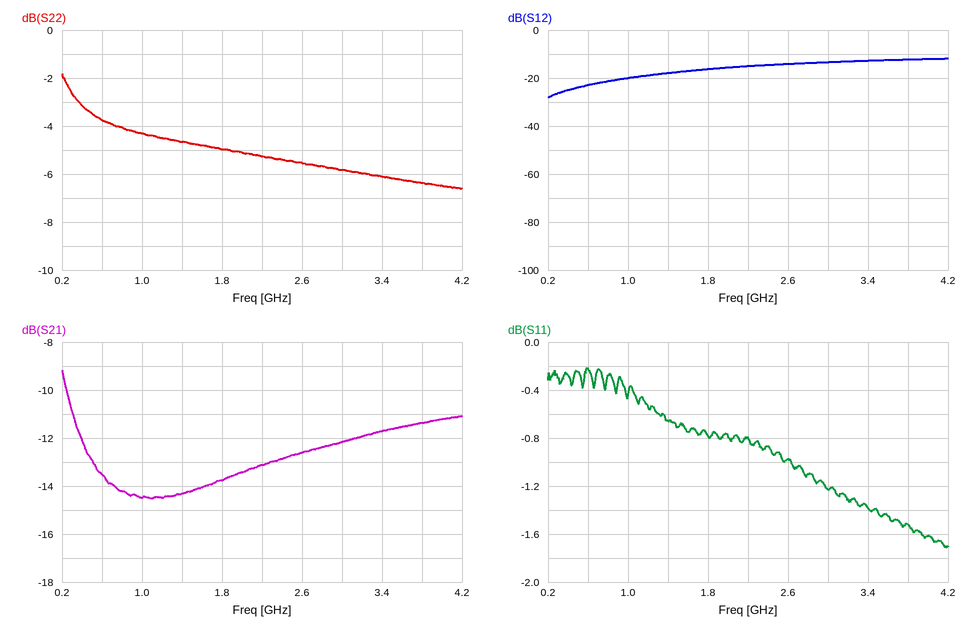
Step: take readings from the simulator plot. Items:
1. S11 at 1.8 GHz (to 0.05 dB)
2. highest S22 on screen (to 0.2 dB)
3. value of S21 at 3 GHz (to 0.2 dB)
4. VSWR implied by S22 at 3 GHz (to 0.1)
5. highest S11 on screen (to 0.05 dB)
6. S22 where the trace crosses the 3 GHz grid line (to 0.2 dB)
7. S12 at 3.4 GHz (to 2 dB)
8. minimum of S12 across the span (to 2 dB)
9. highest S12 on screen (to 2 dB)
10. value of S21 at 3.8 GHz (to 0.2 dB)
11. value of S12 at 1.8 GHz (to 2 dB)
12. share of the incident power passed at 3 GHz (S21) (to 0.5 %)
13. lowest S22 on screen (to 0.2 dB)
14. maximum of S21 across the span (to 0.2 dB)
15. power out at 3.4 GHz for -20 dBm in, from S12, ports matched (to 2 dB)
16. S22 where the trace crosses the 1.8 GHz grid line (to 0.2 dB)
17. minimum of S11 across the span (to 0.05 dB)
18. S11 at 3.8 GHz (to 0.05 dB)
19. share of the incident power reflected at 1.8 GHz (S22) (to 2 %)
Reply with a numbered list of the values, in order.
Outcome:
1. -0.80 dB
2. -1.8 dB
3. -12.2 dB
4. 3.1
5. -0.20 dB
6. -5.8 dB
7. -12 dB
8. -28 dB
9. -12 dB
10. -11.4 dB
11. -16 dB
12. 6.0 %
13. -6.6 dB
14. -9.2 dB
15. -32 dBm
16. -5.0 dB
17. -1.70 dB
18. -1.50 dB
19. 32 %
